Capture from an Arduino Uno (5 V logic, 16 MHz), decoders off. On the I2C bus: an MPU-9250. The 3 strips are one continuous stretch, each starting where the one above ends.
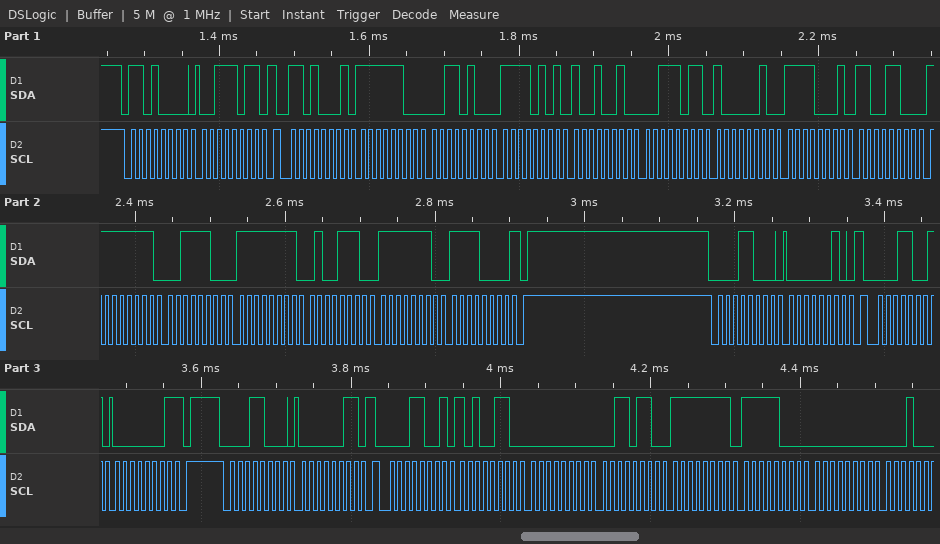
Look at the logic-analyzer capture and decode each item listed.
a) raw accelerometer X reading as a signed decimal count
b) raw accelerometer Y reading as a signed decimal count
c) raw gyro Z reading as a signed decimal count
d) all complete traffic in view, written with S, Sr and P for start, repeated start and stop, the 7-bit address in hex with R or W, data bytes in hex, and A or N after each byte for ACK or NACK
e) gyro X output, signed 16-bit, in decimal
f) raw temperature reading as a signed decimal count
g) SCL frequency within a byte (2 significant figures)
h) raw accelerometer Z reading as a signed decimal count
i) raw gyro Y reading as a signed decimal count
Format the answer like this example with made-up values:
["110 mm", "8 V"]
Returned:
["-972", "-2670", "-272", "S 68W A 3B A Sr 68R A FC A 34 A F5 A 92 A 3B A 82 A F1 A CC A FF A 3C A FF A 4E A FE A F0 N P S 0CW A 02 A Sr 0CR A 01 N P S 0CW A 03 A Sr 0CR A A6 A 00 A 36 A FF A F8 A 00 A", "-196", "-3636", "100 kHz", "15234", "-178"]
